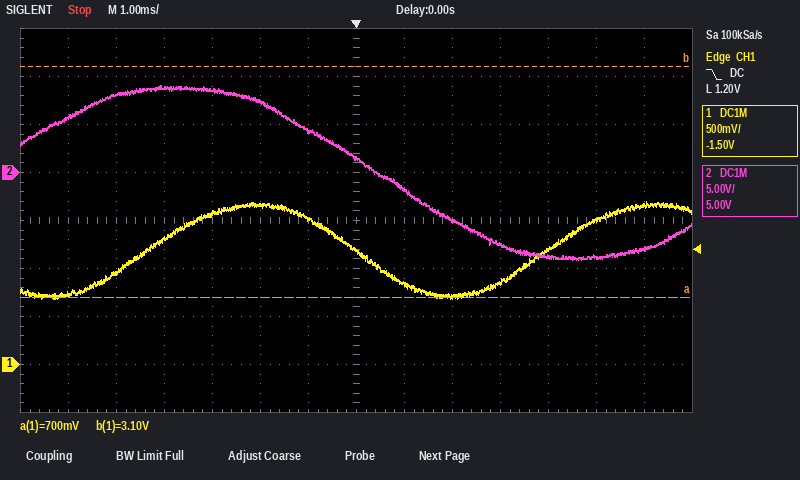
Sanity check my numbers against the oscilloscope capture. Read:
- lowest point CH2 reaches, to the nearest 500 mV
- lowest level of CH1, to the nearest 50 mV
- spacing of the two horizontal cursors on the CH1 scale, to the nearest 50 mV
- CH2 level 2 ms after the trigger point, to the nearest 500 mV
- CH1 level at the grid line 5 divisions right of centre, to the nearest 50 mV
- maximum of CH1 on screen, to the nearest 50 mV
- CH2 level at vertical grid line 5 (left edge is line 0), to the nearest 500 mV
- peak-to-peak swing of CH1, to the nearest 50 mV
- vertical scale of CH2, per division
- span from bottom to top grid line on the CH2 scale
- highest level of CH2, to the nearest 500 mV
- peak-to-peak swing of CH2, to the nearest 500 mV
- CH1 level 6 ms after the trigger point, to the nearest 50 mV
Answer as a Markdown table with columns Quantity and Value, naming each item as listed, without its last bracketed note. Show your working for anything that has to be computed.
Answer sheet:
| Quantity | Value |
|---|---|
| lowest point CH2 reaches, to the nearest 500 mV | -9.0 V |
| lowest level of CH1, to the nearest 50 mV | 700 mV |
| spacing of the two horizontal cursors on the CH1 scale, to the nearest 50 mV | 2.40 V |
| CH2 level 2 ms after the trigger point, to the nearest 500 mV | -5.0 V |
| CH1 level at the grid line 5 divisions right of centre, to the nearest 50 mV | 1.50 V |
| maximum of CH1 on screen, to the nearest 50 mV | 1.70 V |
| CH2 level at vertical grid line 5 (left edge is line 0), to the nearest 500 mV | 7.5 V |
| peak-to-peak swing of CH1, to the nearest 50 mV | 1.70 V − (700 mV) = 1.00 V |
| vertical scale of CH2, per division | 5 V |
| span from bottom to top grid line on the CH2 scale | 40 V |
| highest level of CH2, to the nearest 500 mV | 9.0 V |
| peak-to-peak swing of CH2, to the nearest 500 mV | 9.0 V − (-9.0 V) = 18.0 V |
| CH1 level 6 ms after the trigger point, to the nearest 50 mV | 1.65 V |
